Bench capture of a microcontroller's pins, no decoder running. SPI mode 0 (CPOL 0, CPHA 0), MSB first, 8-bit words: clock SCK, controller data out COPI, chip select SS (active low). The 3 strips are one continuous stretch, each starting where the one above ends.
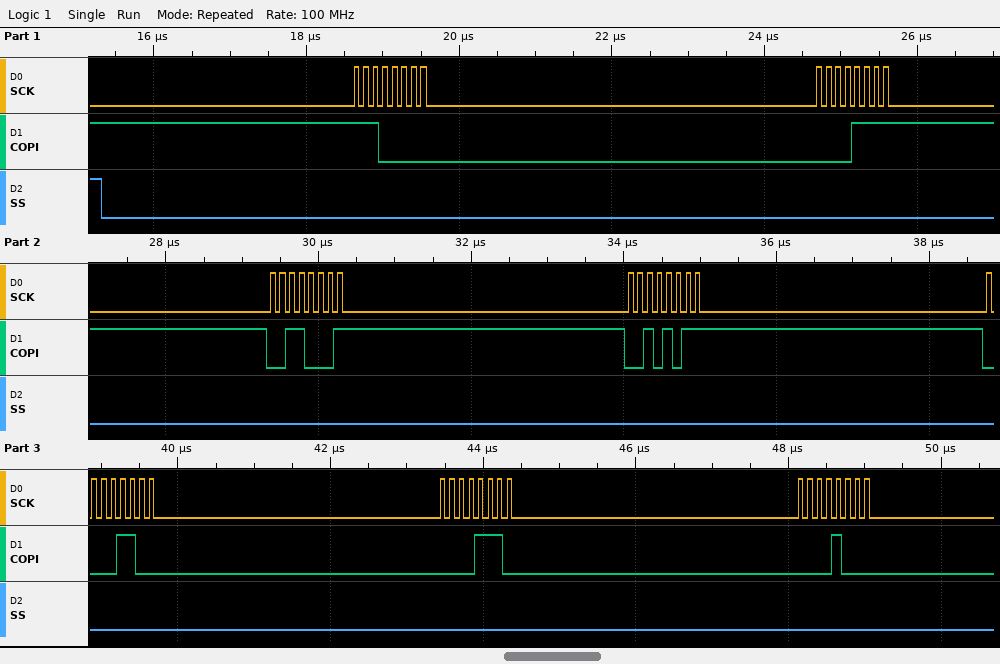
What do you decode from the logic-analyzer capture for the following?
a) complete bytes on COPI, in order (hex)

0xE0 0x0F 0x31 0x2B 0x0C 0x0E 0x08
